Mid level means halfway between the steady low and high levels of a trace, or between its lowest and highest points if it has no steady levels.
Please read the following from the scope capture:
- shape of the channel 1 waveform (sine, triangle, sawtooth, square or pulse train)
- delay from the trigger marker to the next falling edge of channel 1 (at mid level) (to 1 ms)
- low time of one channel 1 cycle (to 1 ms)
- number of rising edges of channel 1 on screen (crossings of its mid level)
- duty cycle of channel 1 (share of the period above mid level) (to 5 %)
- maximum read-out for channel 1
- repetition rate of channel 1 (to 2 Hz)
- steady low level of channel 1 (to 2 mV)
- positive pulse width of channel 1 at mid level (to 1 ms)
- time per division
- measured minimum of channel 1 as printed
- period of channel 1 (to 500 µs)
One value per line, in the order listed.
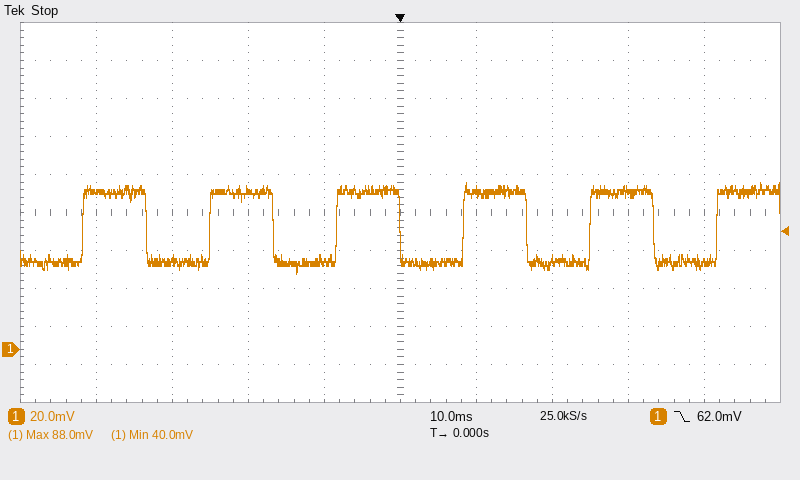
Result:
square
17 ms
8 ms
6
50 %
88.0 mV
60 Hz
46 mV
8 ms
10 ms
40.0 mV
16.5 ms
